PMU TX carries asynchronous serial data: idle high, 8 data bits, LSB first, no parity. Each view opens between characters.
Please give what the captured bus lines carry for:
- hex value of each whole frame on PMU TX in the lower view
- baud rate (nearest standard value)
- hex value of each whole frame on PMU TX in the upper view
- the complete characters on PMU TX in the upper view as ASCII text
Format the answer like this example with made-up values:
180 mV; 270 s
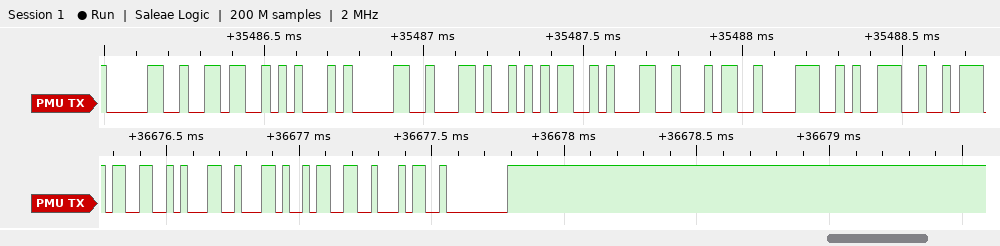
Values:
33, 31, 2C, 33, 34, 00; 38400 baud; 30, 36, 45, 30, 2C, 35, 31, 34, 38, 39; "06E0,51489"
